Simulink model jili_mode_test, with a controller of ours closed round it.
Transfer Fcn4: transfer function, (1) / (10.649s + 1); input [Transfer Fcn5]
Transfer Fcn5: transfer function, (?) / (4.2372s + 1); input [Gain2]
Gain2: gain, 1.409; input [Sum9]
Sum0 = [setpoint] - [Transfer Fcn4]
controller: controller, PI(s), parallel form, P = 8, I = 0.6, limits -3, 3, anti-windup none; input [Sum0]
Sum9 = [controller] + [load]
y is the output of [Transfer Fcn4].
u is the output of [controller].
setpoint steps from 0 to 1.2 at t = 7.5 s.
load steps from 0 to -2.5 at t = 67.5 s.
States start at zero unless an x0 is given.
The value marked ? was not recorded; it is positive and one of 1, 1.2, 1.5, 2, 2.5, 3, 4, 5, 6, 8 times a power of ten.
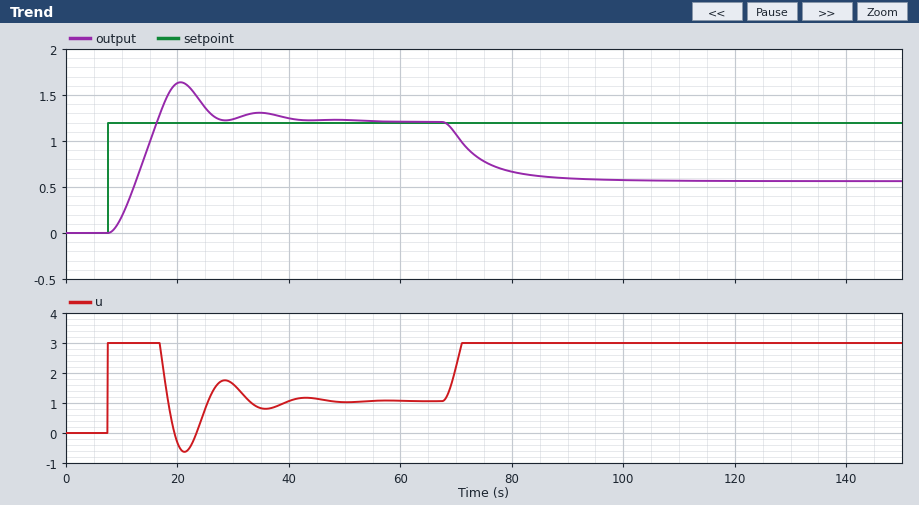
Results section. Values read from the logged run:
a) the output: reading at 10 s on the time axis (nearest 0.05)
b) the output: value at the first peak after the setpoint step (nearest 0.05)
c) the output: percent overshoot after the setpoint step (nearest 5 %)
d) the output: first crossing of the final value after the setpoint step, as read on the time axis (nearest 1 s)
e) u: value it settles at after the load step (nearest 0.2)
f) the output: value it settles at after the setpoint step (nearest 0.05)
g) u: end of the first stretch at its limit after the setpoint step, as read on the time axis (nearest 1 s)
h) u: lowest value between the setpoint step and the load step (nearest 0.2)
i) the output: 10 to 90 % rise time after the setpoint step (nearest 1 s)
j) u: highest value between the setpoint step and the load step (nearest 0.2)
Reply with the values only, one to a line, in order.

0.20
1.65
35 %
16 s
3.0
1.20
17 s
-0.6
6 s
3.0
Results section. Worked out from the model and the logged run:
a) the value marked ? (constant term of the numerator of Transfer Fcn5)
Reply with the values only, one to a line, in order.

0.8
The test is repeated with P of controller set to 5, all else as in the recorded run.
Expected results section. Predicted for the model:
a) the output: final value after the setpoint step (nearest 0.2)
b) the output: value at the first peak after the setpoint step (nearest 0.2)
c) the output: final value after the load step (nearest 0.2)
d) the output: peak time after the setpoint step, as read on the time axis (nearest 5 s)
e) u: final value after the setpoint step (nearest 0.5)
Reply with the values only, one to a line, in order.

1.2
1.8
0.6
20 s
1.0
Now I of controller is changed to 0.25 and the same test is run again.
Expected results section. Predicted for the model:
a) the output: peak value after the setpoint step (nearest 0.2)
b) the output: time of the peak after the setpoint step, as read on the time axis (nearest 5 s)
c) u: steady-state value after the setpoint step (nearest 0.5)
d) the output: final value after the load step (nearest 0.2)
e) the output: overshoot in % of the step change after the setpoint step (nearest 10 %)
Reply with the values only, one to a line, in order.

1.4
20 s
1.0
0.6
20 %
